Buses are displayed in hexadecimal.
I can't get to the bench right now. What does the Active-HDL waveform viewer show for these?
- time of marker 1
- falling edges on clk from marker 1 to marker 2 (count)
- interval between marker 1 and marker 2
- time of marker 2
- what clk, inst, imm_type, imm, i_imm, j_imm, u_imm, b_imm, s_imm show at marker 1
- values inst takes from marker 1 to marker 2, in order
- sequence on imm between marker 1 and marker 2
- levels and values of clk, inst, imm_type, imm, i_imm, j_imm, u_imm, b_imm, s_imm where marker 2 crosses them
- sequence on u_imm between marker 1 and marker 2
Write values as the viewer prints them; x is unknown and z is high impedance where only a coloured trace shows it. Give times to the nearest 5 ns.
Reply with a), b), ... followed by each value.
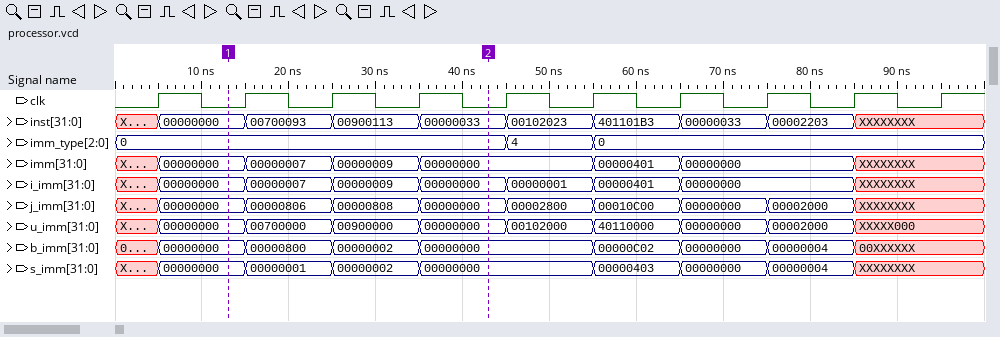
a) 15 ns
b) 3
c) 30 ns
d) 45 ns
e) clk=0, inst=00000000, imm_type=0, imm=00000000, i_imm=00000000, j_imm=00000000, u_imm=00000000, b_imm=00000000, s_imm=00000000
f) 00000000, 00700093, 00900113, 00000033
g) 00000000, 00000007, 00000009, 00000000
h) clk=0, inst=00000033, imm_type=0, imm=00000000, i_imm=00000000, j_imm=00000000, u_imm=00000000, b_imm=00000000, s_imm=00000000
i) 00000000, 00700000, 00900000, 00000000
